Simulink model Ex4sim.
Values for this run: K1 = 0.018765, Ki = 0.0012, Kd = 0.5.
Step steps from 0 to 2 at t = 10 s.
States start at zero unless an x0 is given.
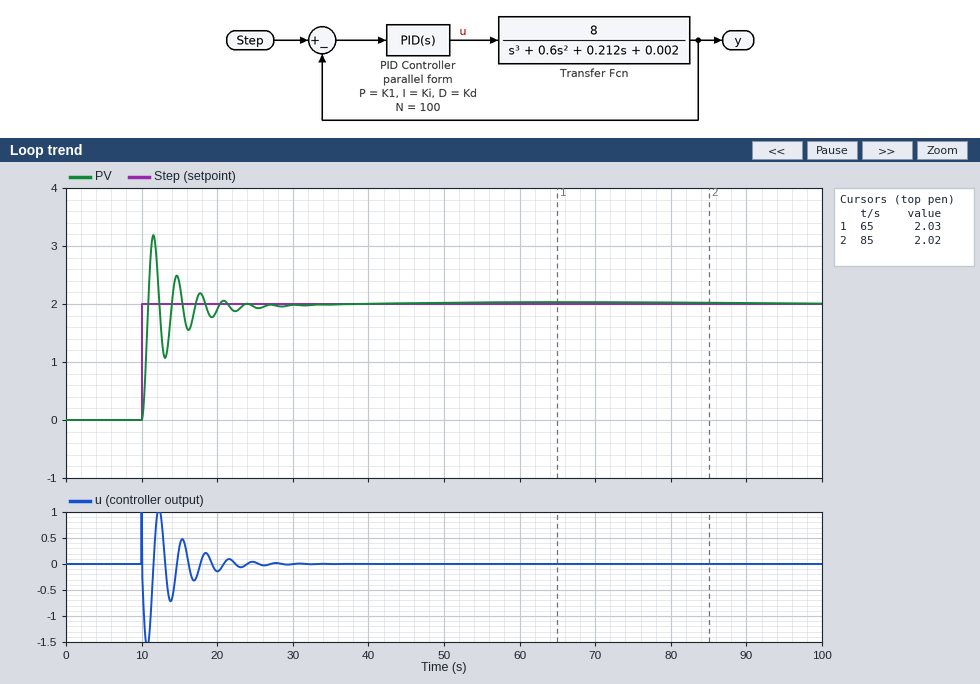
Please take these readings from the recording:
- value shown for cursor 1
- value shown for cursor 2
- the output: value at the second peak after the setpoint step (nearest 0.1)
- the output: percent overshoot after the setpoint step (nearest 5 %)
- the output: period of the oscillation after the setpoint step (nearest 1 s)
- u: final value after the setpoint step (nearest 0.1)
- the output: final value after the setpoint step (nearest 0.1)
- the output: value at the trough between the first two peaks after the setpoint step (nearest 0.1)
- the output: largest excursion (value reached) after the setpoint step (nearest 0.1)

2.03
2.02
2.5
60 %
3 s
0.0
2.0
1.1
3.2
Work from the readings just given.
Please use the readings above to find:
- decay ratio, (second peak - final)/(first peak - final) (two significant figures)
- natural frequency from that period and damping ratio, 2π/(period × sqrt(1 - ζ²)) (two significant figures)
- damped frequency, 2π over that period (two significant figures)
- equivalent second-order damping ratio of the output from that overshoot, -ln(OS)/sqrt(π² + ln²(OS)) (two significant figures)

0.42
2.1 rad/s
2.1 rad/s
0.16
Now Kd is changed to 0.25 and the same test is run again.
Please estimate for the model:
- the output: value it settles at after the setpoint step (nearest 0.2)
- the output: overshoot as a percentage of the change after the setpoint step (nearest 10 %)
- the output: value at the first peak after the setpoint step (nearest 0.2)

2.0
50 %
3.0
